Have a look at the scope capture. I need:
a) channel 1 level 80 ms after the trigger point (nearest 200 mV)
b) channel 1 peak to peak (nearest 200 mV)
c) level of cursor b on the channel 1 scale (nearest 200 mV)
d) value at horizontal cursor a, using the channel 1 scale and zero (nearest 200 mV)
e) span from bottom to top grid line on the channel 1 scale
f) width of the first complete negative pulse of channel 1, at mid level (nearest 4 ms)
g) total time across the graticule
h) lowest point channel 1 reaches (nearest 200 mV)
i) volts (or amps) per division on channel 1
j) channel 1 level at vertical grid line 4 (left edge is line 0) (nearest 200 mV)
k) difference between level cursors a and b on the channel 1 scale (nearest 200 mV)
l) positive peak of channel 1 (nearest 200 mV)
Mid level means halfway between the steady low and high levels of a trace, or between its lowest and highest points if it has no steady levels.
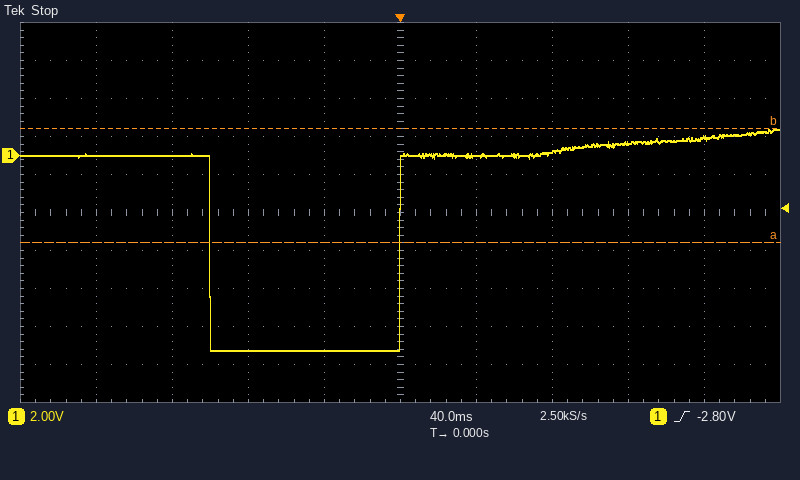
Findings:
200 mV
11.6 V
1.4 V
-4.6 V
20 V
100 ms
400 ms
-10.2 V
2 V
-10.2 V
6.0 V
1.4 V
